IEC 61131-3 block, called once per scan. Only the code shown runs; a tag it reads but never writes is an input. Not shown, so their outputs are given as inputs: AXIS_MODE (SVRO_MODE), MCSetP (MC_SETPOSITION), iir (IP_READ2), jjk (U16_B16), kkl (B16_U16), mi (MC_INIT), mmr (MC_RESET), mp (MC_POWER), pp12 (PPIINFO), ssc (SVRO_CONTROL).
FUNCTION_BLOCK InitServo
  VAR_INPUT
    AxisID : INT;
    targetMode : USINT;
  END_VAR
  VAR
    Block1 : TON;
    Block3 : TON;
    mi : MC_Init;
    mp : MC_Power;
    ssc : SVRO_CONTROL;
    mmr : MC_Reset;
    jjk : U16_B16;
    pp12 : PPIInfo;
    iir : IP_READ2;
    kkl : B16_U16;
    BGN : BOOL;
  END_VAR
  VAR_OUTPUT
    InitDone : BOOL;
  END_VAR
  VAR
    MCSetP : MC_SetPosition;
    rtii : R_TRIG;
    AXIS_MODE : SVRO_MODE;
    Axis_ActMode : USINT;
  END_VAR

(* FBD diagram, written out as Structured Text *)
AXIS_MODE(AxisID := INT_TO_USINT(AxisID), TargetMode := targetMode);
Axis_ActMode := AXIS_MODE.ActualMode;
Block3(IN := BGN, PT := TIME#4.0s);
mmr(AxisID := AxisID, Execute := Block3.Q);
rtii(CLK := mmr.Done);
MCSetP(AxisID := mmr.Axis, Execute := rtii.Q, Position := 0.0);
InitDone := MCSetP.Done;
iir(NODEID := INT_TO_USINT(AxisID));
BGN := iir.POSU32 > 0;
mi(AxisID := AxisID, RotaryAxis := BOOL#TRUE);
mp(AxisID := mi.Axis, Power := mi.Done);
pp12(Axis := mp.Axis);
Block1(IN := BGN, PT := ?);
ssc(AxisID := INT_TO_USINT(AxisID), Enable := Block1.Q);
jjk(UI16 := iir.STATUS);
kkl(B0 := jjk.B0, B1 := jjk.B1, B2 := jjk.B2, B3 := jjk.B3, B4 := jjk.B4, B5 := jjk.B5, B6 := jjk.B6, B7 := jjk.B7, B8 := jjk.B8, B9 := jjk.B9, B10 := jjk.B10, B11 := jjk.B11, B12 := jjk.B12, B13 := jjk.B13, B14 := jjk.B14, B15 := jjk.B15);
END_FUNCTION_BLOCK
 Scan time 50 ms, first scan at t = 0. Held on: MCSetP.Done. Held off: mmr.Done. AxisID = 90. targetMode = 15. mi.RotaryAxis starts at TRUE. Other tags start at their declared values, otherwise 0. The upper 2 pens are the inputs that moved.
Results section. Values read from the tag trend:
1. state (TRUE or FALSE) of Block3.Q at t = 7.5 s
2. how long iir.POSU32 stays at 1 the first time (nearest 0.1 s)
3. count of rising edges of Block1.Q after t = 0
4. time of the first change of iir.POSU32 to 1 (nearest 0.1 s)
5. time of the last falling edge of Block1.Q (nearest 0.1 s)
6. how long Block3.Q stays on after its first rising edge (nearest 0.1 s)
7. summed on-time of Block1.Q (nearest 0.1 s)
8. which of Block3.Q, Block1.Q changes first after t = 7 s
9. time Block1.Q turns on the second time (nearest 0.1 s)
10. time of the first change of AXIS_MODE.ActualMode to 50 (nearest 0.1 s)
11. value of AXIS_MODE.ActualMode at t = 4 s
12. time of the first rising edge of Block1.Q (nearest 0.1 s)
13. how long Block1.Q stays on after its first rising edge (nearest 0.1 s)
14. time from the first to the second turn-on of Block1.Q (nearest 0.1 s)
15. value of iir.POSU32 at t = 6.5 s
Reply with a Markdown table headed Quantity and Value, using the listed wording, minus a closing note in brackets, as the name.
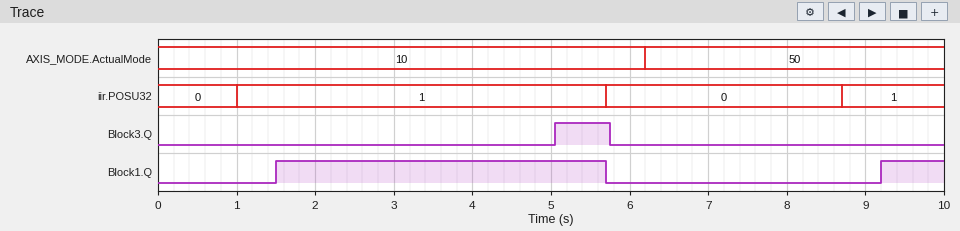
| Quantity | Value |
|---|---|
| state (TRUE or FALSE) of Block3.Q at t = 7.5 s | FALSE |
| how long iir.POSU32 stays at 1 the first time | 4.7 s |
| count of rising edges of Block1.Q after t = 0 | 2 |
| time of the first change of iir.POSU32 to 1 | 1.0 s |
| time of the last falling edge of Block1.Q | 5.7 s |
| how long Block3.Q stays on after its first rising edge | 0.7 s |
| summed on-time of Block1.Q | 5.0 s |
| which of Block3.Q, Block1.Q changes first after t = 7 s | Block1.Q |
| time Block1.Q turns on the second time | 9.2 s |
| time of the first change of AXIS_MODE.ActualMode to 50 | 6.2 s |
| value of AXIS_MODE.ActualMode at t = 4 s | 10 |
| time of the first rising edge of Block1.Q | 1.5 s |
| how long Block1.Q stays on after its first rising edge | 4.2 s |
| time from the first to the second turn-on of Block1.Q | 7.7 s |
| value of iir.POSU32 at t = 6.5 s | 0 |
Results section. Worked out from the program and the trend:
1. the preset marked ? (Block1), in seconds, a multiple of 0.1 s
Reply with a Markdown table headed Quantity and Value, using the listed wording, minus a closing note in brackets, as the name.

| Quantity | Value |
|---|---|
| the preset marked ? (Block1), in seconds, a multiple of 0.1 s | 0.5 s |
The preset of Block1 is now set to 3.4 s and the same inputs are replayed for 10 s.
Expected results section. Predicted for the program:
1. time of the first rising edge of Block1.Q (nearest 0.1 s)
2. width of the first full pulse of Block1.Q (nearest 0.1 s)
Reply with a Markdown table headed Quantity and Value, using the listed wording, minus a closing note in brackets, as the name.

| Quantity | Value |
|---|---|
| time of the first rising edge of Block1.Q | 4.4 s |
| width of the first full pulse of Block1.Q | 1.3 s |
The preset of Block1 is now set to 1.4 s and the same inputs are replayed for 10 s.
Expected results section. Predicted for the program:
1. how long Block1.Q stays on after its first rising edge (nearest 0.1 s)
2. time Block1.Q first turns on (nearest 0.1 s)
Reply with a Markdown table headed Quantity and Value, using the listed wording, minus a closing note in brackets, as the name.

| Quantity | Value |
|---|---|
| how long Block1.Q stays on after its first rising edge | 3.3 s |
| time Block1.Q first turns on | 2.4 s |
